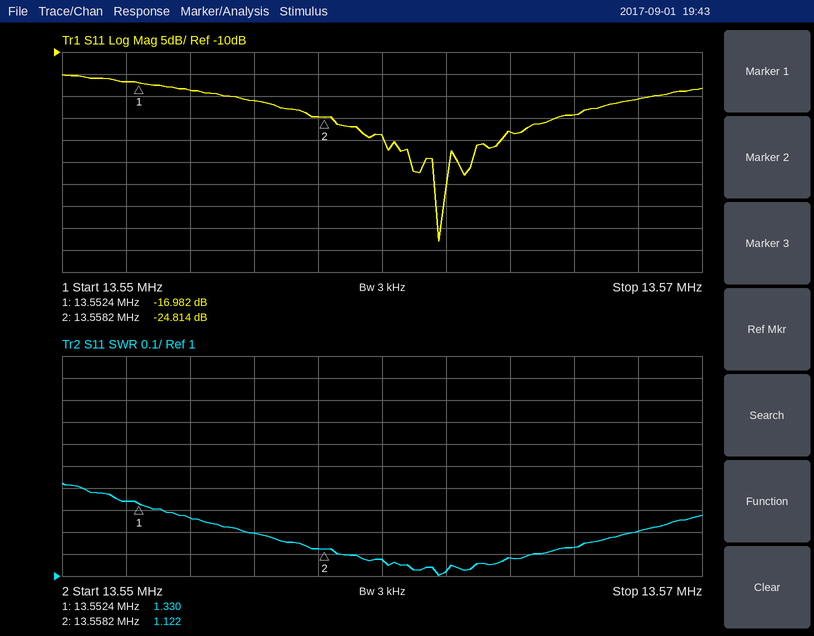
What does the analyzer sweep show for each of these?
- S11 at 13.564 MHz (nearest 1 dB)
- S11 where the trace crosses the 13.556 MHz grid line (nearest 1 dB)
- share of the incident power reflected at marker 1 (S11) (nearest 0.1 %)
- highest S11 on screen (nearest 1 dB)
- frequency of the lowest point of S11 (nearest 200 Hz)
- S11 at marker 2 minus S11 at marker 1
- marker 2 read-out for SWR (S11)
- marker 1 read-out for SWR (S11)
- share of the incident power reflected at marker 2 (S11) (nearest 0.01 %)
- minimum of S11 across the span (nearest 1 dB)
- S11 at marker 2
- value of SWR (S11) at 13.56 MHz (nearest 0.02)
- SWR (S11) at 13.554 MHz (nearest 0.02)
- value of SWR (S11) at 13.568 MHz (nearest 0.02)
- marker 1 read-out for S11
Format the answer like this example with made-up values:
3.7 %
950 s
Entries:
-28 dB
-21 dB
2.0 %
-15 dB
13.5618 MHz
-7.832 dB
1.122
1.330
0.33 %
-53 dB
-24.814 dB
1.08
1.26
1.20
-16.982 dB
